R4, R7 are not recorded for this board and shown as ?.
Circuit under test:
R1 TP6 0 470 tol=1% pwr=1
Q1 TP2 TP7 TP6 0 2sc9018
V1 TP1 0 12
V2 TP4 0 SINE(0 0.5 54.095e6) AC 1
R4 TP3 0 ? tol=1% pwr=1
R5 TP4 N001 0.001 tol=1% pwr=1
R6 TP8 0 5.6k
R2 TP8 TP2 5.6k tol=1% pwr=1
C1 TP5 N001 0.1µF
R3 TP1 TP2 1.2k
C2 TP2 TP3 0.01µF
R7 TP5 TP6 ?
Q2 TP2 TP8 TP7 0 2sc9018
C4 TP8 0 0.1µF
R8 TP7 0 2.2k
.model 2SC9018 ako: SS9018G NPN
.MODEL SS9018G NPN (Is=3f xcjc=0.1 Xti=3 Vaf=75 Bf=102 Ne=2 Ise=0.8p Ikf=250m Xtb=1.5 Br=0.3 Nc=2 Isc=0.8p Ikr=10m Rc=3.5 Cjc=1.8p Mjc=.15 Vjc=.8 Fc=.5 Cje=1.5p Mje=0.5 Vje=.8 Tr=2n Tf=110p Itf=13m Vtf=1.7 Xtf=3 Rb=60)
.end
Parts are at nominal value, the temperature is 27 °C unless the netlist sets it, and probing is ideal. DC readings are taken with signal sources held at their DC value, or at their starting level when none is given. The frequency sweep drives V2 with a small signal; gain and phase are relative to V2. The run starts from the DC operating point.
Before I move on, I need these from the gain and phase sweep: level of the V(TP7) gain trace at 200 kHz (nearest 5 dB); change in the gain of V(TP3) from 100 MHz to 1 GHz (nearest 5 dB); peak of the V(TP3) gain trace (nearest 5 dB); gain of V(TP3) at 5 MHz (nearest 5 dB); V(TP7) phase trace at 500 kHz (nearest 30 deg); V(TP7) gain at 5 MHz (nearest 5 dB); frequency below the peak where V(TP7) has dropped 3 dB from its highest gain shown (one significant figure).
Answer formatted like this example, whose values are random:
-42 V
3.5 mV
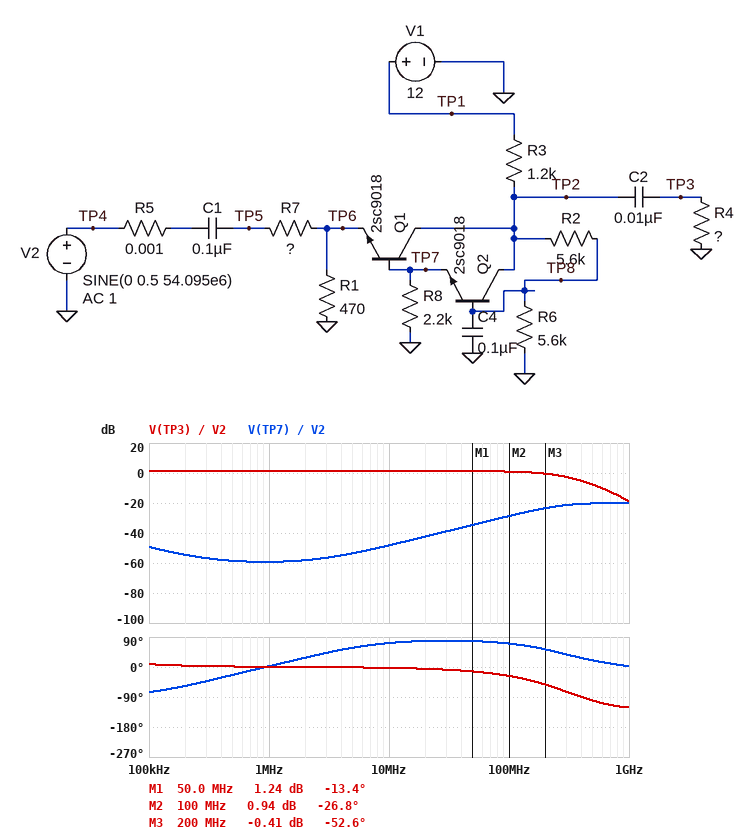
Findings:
-55 dB
-20 dB
0 dB
0 dB
-30 deg
-55 dB
200 MHz
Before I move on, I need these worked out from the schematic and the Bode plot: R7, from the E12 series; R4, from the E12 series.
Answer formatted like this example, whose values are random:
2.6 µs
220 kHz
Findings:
330 Ω
680 Ω
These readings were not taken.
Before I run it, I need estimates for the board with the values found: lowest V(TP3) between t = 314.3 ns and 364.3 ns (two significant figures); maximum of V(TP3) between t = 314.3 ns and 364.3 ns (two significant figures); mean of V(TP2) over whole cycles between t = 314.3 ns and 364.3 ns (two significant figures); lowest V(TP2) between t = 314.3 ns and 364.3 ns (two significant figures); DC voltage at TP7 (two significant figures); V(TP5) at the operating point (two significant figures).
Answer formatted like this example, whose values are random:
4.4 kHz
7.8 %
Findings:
-580 mV
570 mV
6.0 V
5.5 V
2.3 V
1.6 V
